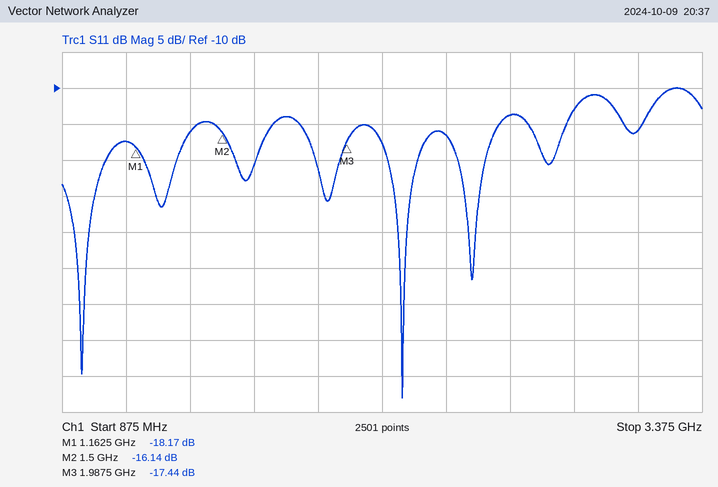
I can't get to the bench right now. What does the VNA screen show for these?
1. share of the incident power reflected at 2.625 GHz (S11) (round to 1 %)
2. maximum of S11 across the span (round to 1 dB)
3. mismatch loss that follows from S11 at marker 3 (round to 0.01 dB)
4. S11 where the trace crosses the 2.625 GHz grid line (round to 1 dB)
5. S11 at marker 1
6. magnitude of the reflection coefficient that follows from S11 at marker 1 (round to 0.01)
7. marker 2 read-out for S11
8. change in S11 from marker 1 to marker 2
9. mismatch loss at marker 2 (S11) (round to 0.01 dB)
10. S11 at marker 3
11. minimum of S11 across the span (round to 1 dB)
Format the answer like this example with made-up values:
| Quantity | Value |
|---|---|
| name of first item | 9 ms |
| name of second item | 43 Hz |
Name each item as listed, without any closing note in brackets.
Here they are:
| Quantity | Value |
|---|---|
| share of the incident power reflected at 2.625 GHz (S11) | 4 % |
| maximum of S11 across the span | -10 dB |
| mismatch loss that follows from S11 at marker 3 | 0.08 dB |
| S11 where the trace crosses the 2.625 GHz grid line | -14 dB |
| S11 at marker 1 | -18.17 dB |
| magnitude of the reflection coefficient that follows from S11 at marker 1 | 0.12 |
| marker 2 read-out for S11 | -16.14 dB |
| change in S11 from marker 1 to marker 2 | 2.03 dB |
| mismatch loss at marker 2 (S11) | 0.11 dB |
| S11 at marker 3 | -17.44 dB |
| minimum of S11 across the span | -53 dB |
